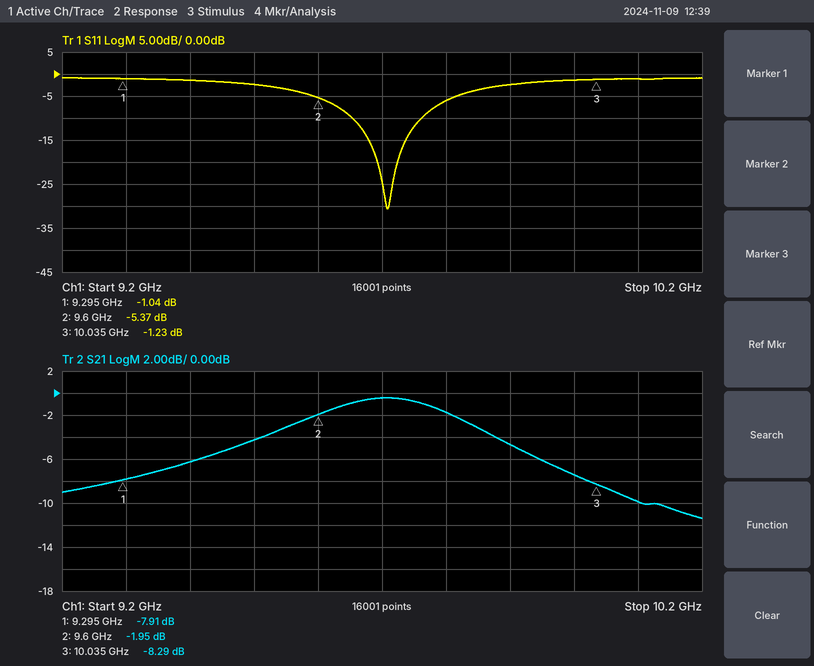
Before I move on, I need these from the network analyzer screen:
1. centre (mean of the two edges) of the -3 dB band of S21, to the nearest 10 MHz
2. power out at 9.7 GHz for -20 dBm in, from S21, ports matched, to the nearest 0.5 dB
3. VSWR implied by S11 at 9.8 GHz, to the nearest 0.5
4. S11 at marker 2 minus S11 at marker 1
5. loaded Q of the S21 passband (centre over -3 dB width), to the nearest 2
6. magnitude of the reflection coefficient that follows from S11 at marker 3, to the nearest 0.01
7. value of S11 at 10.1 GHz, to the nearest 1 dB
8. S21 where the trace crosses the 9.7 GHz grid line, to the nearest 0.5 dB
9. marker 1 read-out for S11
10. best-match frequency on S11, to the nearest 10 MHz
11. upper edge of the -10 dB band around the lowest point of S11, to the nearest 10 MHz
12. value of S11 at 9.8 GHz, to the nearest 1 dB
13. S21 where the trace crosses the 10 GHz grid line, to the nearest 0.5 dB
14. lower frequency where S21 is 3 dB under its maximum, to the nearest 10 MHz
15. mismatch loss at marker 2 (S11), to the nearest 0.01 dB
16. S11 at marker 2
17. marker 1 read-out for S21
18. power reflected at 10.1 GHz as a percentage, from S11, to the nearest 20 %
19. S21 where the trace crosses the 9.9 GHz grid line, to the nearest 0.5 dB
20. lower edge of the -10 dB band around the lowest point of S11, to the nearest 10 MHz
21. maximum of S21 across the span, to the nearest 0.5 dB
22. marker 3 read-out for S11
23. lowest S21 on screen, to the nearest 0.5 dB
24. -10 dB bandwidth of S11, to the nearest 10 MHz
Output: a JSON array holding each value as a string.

["9.70 GHz", "-20.5 dBm", "3.0", "-4.33 dB", "30", "0.87", "-1 dB", "-0.5 dB", "-1.04 dB", "9.71 GHz", "9.76 GHz", "-6 dB", "-7.5 dB", "9.54 GHz", "1.49 dB", "-5.37 dB", "-7.91 dB", "80 %", "-4.5 dB", "9.65 GHz", "-0.5 dB", "-1.23 dB", "-11.5 dB", "110 MHz"]
